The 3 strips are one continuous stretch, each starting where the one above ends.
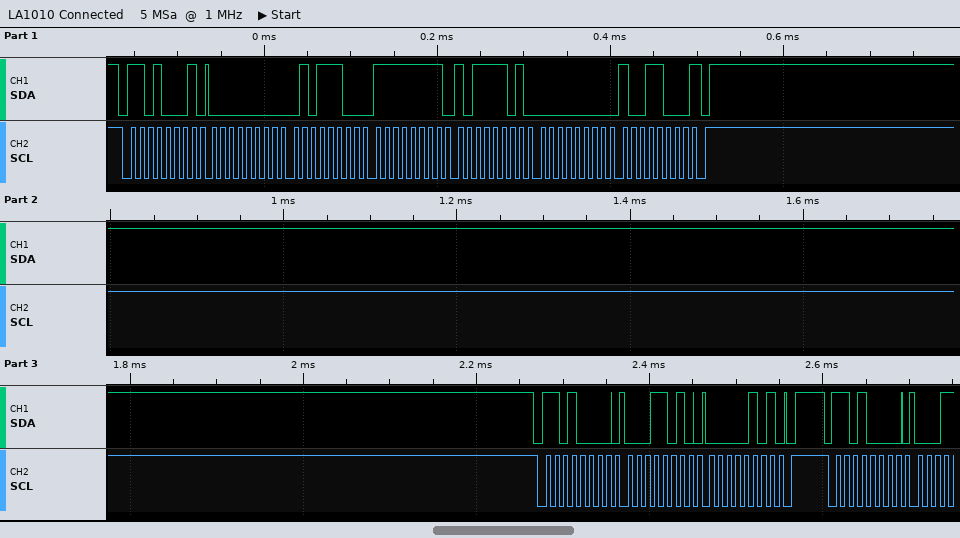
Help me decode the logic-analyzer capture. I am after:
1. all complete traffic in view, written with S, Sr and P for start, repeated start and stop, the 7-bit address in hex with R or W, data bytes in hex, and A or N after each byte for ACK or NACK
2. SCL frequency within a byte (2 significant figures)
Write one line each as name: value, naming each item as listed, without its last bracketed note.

all complete traffic in view, written with S, Sr and P for start, repeated start and stop, the 7-bit address in hex with R or W, data bytes in hex, and A or N after each byte for ACK or NACK: S 68R A 00 A 5C A FF A BD A 00 A 98 N P S 68W A 1A A 05 A P S 68W A
SCL frequency within a byte: 100 kHz
